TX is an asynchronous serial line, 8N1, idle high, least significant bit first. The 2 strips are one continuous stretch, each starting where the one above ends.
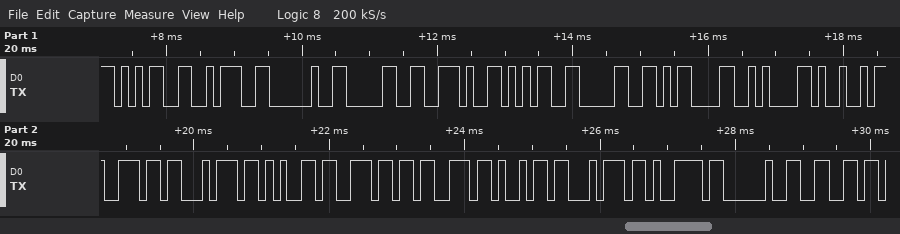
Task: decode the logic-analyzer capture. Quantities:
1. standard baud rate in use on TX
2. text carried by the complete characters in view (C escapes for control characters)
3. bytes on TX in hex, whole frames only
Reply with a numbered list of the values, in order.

1. 9600 baud
2. "5: 0.50\r\nIntensity f"
3. 0x35 0x3A 0x20 0x30 0x2E 0x35 0x30 0x0D 0x0A 0x49 0x6E 0x74 0x65 0x6E 0x73 0x69 0x74 0x79 0x20 0x66
